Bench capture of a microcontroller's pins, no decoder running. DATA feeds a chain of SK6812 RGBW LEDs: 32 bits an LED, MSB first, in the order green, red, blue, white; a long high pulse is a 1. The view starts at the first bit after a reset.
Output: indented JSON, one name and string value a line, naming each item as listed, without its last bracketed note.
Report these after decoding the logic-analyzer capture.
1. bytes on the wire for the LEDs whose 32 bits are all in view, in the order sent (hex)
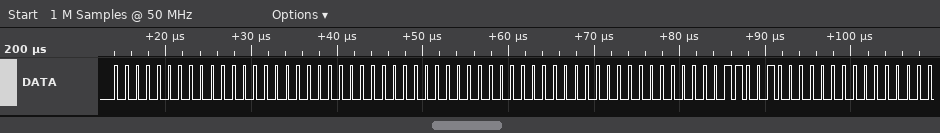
{
  "bytes on the wire for the LEDs whose 32 bits are all in view, in the order sent": "00 00 00 00 00 00 00 64"
}
